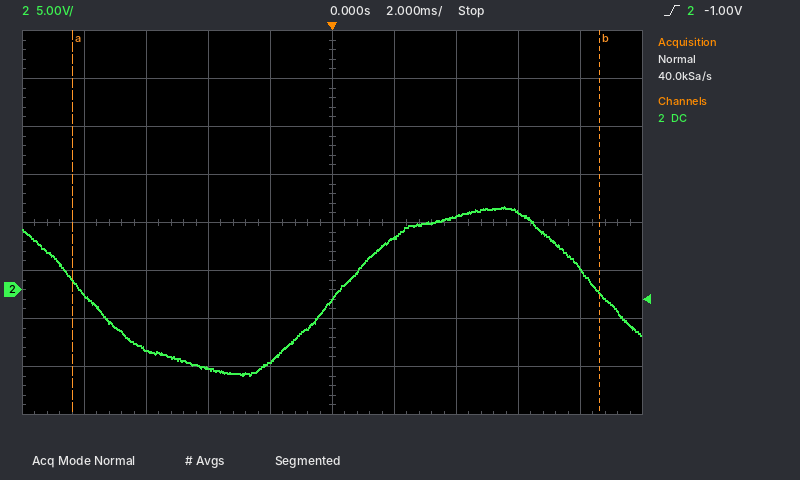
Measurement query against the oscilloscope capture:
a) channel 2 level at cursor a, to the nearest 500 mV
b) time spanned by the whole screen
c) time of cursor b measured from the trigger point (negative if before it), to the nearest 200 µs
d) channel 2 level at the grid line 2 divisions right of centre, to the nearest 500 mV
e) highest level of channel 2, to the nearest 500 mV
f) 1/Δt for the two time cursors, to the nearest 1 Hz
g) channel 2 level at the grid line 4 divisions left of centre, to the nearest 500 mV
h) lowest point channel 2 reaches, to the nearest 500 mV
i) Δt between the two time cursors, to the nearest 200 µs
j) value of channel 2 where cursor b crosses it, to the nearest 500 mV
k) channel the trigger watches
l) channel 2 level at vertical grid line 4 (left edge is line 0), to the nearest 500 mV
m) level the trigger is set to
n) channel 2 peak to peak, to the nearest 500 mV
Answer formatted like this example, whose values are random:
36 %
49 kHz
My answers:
1.0 V
20 ms
+8.6 ms
7.5 V
8.5 V
59 Hz
-500 mV
-9.0 V
17.0 ms
-500 mV
channel 2
-7.5 V
-1.00 V
17.5 V
